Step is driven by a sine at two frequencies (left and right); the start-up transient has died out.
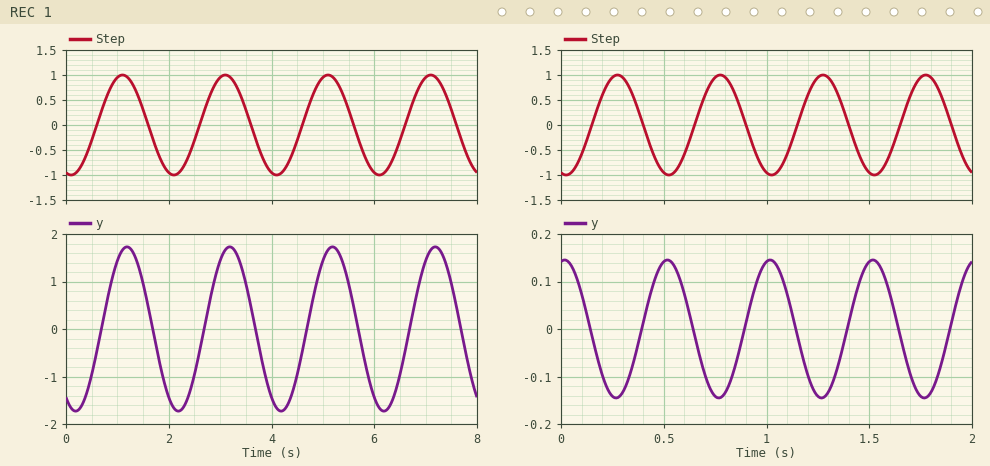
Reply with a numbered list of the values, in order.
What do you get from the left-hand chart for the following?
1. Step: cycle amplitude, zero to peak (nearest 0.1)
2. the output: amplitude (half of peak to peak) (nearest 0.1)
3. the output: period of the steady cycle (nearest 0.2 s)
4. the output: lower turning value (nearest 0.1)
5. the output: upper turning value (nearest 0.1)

1. 1.0
2. 1.7
3. 2.0 s
4. -1.7
5. 1.7
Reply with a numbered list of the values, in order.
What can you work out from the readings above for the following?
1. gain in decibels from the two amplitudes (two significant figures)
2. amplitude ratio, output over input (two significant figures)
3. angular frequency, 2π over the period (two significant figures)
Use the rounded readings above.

1. 4.6 dB
2. 1.7
3. 3.1 rad/s
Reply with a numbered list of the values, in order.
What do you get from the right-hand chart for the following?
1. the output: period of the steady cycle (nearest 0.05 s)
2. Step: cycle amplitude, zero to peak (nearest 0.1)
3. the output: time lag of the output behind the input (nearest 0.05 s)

1. 0.50 s
2. 1.0
3. 0.25 s
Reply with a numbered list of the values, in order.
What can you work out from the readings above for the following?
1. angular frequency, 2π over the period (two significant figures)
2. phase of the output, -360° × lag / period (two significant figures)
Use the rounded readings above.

1. 13 rad/s
2. -180°
